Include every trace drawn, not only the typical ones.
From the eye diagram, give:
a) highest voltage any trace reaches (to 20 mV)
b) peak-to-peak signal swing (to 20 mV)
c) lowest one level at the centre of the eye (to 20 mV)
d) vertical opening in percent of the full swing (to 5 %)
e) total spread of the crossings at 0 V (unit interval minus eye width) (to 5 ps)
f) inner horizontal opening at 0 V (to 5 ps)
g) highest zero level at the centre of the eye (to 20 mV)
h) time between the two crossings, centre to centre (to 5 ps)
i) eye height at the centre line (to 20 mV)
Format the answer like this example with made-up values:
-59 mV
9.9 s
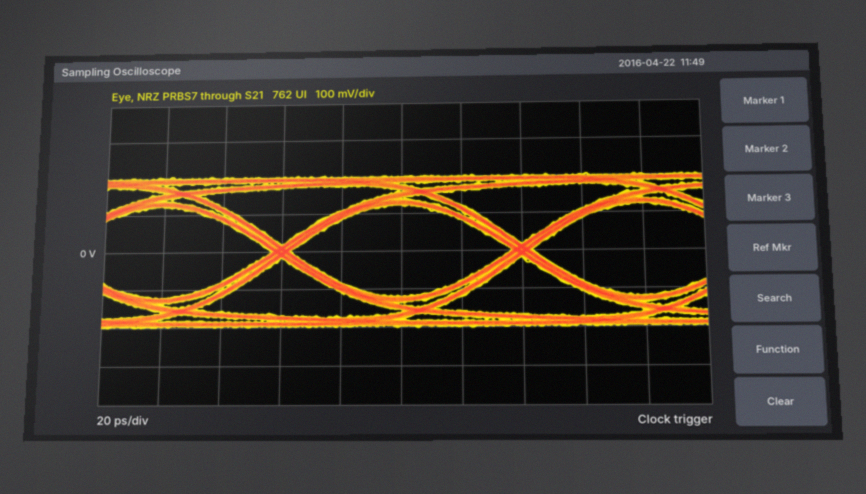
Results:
200 mV
400 mV
120 mV
60 %
5 ps
75 ps
-120 mV
80 ps
240 mV
